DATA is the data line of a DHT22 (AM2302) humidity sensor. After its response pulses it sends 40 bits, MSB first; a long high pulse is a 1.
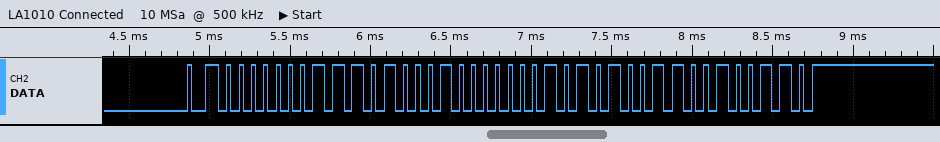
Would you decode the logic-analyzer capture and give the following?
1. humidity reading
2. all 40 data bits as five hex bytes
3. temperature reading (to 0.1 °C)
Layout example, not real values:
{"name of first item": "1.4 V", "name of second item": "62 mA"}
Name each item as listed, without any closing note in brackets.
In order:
{"humidity reading": "46.5 %", "all 40 data bits as five hex bytes": "01 D1 01 53 26", "temperature reading": "33.9 °C"}
